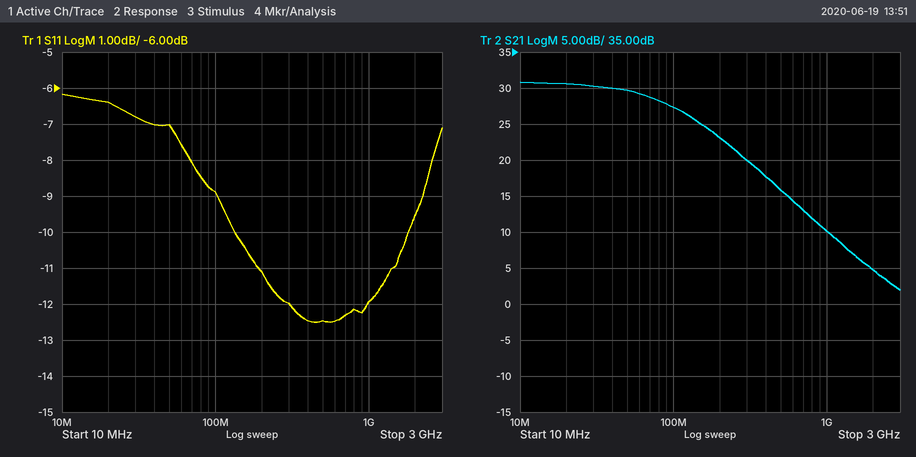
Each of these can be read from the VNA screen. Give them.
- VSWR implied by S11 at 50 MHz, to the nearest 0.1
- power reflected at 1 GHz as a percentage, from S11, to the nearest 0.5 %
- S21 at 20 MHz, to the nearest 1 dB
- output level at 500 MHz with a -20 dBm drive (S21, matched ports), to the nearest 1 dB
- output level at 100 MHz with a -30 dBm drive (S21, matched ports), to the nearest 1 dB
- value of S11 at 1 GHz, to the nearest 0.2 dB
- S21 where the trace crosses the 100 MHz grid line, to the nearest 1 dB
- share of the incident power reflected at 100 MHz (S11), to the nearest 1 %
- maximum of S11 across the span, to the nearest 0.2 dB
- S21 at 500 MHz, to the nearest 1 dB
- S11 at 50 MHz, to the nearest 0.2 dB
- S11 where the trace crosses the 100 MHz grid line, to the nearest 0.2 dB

2.6
6.5 %
31 dB
-4 dBm
-3 dBm
-12.0 dB
27 dB
13 %
-6.2 dB
16 dB
-7.0 dB
-8.8 dB
